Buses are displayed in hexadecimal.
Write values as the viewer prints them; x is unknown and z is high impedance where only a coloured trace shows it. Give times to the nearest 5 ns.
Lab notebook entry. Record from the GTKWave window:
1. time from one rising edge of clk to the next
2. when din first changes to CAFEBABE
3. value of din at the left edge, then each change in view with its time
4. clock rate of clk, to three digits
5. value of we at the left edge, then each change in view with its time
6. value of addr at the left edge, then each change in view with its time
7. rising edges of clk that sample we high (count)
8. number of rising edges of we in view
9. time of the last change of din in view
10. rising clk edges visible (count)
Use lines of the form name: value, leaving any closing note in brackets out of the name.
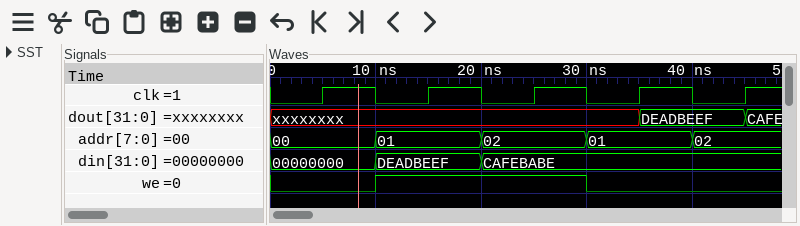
time from one rising edge of clk to the next: 10 ns
when din first changes to CAFEBABE: 20 ns
value of din at the left edge, then each change in view with its time: 00000000, DEADBEEF at 10 ns, CAFEBABE at 20 ns
clock rate of clk, to three digits: 100 MHz
value of we at the left edge, then each change in view with its time: 0, 1 at 10 ns, 0 at 30 ns
value of addr at the left edge, then each change in view with its time: 00, 01 at 10 ns, 02 at 20 ns, 01 at 30 ns, 02 at 40 ns
rising edges of clk that sample we high: 2
number of rising edges of we in view: 1
time of the last change of din in view: 20 ns
rising clk edges visible: 5
